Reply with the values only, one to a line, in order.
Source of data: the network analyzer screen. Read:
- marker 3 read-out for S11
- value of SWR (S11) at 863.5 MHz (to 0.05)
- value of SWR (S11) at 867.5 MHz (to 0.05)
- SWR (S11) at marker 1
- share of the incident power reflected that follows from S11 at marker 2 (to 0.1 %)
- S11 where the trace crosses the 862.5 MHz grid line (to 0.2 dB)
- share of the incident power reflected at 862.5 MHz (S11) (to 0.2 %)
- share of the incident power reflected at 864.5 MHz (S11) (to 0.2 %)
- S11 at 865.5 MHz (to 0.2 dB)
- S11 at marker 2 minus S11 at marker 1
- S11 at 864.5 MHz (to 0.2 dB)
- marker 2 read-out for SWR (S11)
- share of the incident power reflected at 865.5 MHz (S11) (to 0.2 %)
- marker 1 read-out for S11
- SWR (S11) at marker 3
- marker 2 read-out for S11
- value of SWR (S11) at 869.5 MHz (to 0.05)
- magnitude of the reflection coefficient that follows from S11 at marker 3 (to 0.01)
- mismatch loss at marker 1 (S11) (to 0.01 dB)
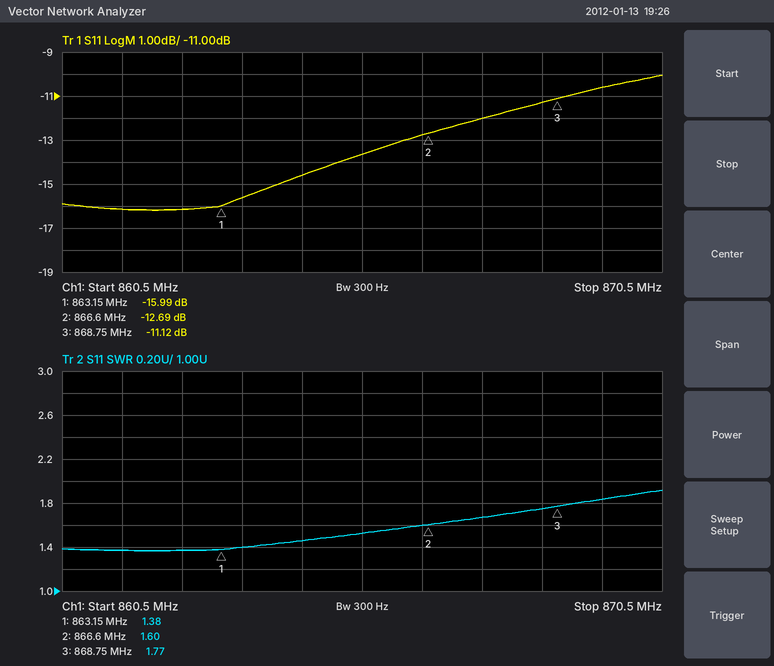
-11.12 dB
1.40
1.65
1.38
5.4 %
-16.2 dB
2.4 %
3.4 %
-13.6 dB
3.30 dB
-14.6 dB
1.60
4.4 %
-15.99 dB
1.77
-12.69 dB
1.85
0.28
0.11 dB
